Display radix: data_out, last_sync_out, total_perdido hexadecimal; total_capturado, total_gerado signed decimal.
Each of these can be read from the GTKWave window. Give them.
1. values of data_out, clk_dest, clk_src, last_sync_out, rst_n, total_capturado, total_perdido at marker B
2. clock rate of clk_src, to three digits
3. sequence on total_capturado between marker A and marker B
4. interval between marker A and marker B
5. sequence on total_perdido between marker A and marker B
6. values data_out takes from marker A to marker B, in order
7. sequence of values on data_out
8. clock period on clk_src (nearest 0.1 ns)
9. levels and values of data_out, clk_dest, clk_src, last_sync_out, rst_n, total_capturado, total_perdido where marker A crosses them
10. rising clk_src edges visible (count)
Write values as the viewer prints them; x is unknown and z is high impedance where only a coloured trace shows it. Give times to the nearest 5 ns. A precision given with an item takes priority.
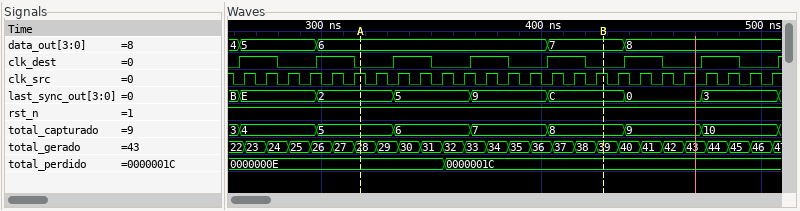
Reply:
data_out=7, clk_dest=0, clk_src=1, last_sync_out=C, rst_n=1, total_capturado=8, total_perdido=0000001C
100 MHz
5, 6, 7, 8
110 ns
0000000E, 0000001C
6, 7
4, 5, 6, 7, 8
10 ns
data_out=6, clk_dest=0, clk_src=1, last_sync_out=2, rst_n=1, total_capturado=5, total_perdido=0000000E
25
